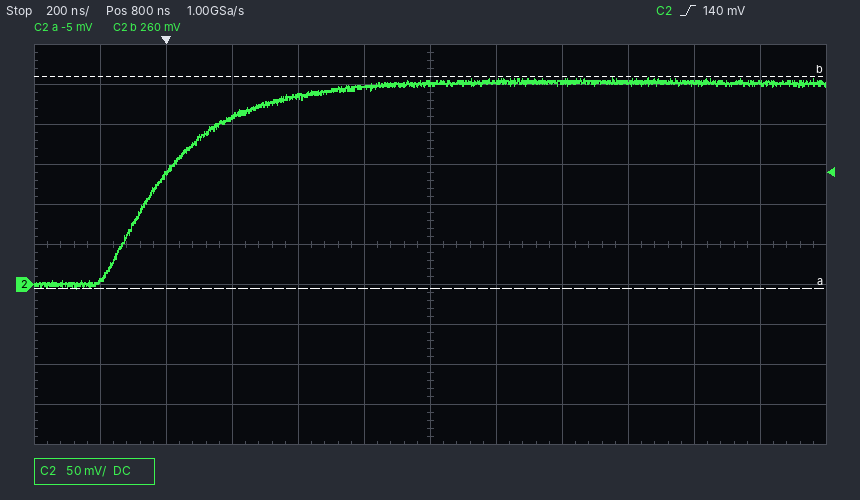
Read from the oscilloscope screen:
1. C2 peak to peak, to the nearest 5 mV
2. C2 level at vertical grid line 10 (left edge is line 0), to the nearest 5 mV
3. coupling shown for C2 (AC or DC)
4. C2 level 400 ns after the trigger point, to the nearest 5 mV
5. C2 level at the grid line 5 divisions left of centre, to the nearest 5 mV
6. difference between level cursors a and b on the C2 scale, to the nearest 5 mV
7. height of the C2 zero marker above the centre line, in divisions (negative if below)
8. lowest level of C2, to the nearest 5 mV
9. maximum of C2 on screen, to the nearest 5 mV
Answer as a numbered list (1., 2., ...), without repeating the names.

1. 265 mV
2. 250 mV
3. DC
4. 235 mV
5. 5 mV
6. 265 mV
7. -1.0 div
8. -5 mV
9. 260 mV
